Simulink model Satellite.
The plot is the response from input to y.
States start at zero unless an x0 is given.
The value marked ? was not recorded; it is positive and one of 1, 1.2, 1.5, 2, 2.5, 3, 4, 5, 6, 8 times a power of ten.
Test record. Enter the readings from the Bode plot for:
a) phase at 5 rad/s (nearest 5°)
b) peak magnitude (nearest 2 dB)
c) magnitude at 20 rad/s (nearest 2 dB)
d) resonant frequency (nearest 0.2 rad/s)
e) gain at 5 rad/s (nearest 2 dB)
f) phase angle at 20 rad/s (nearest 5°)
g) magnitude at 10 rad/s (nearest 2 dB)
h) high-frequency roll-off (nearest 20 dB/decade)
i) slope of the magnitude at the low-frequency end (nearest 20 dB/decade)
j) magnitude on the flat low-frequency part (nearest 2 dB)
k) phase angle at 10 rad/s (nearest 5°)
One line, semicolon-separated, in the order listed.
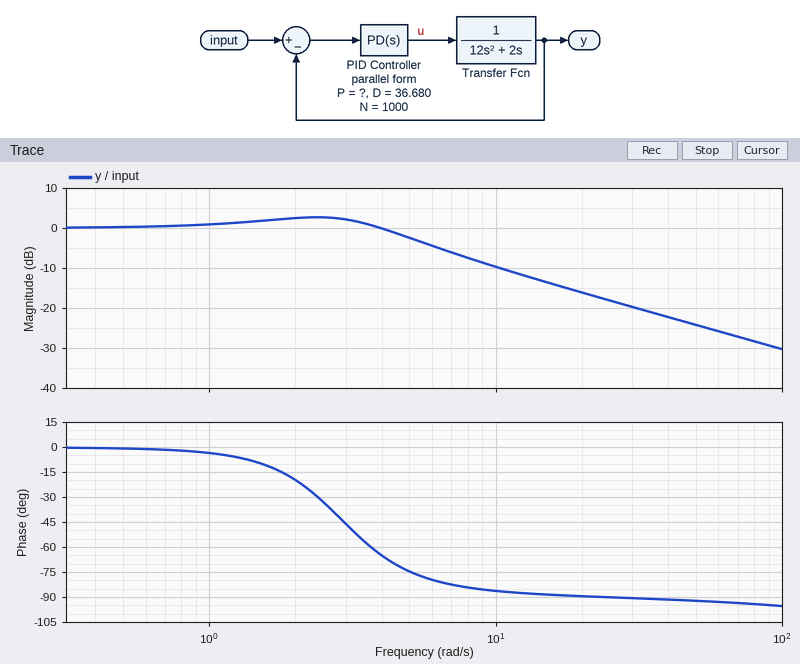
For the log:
-75°; 2 dB; -16 dB; 2.4 rad/s; -2 dB; -90°; -10 dB; -20 dB/decade; 0 dB/decade; 0 dB; -85°
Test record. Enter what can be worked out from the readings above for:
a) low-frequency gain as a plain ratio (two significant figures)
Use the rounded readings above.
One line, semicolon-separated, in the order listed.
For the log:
1.0
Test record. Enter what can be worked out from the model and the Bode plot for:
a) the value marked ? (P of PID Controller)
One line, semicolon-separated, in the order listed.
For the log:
100
